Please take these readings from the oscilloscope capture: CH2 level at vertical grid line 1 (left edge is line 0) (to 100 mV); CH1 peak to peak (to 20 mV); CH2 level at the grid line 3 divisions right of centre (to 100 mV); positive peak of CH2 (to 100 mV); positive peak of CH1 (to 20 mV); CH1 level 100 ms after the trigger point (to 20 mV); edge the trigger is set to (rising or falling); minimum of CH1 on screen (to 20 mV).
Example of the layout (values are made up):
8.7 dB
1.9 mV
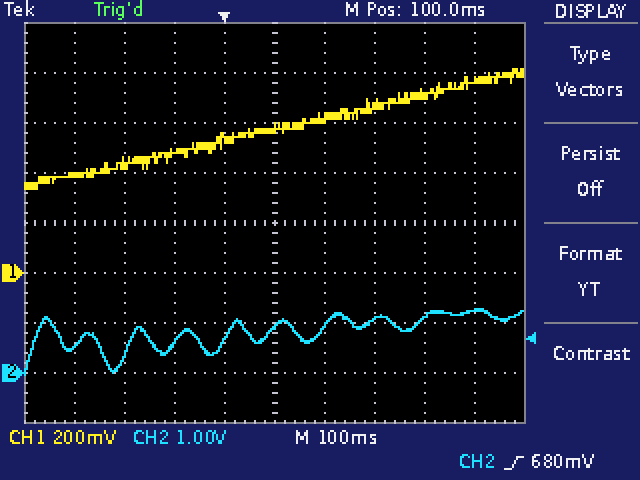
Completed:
500 mV
480 mV
1.1 V
1.3 V
820 mV
580 mV
rising
340 mV
